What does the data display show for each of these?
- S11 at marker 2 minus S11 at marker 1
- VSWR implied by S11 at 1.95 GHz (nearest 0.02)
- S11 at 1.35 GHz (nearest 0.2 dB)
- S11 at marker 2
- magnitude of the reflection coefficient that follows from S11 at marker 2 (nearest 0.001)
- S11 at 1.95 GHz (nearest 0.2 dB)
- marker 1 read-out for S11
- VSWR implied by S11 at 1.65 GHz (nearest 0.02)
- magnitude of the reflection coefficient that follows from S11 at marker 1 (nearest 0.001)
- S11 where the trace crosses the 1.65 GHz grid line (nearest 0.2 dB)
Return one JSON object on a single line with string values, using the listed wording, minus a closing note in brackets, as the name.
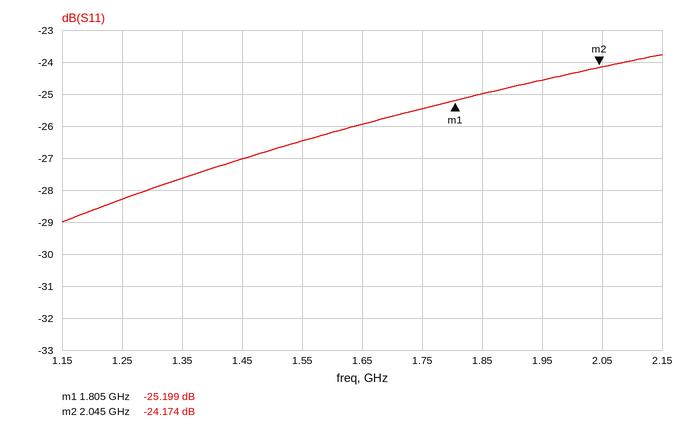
{"S11 at marker 2 minus S11 at marker 1": "1.025 dB", "VSWR implied by S11 at 1.95 GHz": "1.12", "S11 at 1.35 GHz": "-27.6 dB", "S11 at marker 2": "-24.174 dB", "magnitude of the reflection coefficient that follows from S11 at marker 2": "0.062", "S11 at 1.95 GHz": "-24.6 dB", "marker 1 read-out for S11": "-25.199 dB", "VSWR implied by S11 at 1.65 GHz": "1.10", "magnitude of the reflection coefficient that follows from S11 at marker 1": "0.055", "S11 where the trace crosses the 1.65 GHz grid line": "-26.0 dB"}
